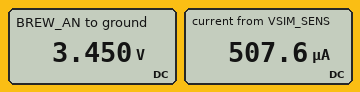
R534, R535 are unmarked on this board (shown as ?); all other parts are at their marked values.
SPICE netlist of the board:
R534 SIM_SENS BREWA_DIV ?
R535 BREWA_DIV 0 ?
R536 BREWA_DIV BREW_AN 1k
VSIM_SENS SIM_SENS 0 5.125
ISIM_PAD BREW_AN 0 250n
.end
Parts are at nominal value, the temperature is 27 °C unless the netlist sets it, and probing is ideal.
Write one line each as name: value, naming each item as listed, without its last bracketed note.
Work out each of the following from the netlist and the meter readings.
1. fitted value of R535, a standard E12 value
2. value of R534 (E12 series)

fitted value of R535, a standard E12 value: 6.8 kΩ
value of R534: 3.3 kΩ
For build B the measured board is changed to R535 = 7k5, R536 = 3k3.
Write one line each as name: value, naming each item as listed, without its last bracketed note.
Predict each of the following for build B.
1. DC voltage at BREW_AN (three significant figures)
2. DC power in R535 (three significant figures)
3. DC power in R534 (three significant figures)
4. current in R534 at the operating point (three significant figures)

DC voltage at BREW_AN: 3.56 V
DC power in R535: 1.69 mW
DC power in R534: 744 µW
current in R534 at the operating point: 475 µA
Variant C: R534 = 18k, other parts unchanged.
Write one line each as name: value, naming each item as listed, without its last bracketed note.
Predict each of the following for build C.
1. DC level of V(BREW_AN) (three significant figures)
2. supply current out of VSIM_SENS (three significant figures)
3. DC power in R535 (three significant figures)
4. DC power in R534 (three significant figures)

DC level of V(BREW_AN): 1.40 V
supply current out of VSIM_SENS: 207 µA
DC power in R535: 290 µW
DC power in R534: 769 µW
